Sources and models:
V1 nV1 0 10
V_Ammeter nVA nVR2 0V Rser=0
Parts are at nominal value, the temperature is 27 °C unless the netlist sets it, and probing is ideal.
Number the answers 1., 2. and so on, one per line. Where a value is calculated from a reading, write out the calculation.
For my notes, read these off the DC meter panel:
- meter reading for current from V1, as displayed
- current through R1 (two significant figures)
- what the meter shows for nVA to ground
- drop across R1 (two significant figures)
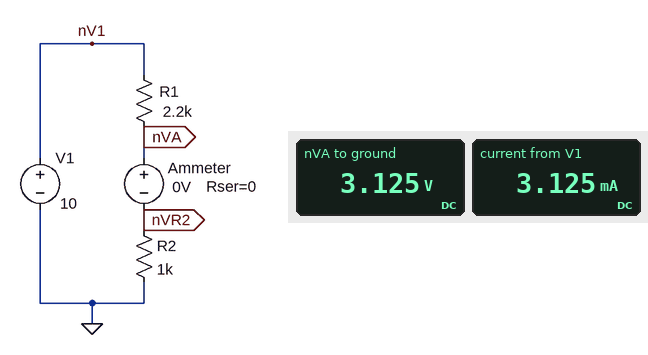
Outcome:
1. 3.125 mA
2. (10 V - 3.125 V) / 2.2 kΩ = 3.1 mA
3. 3.125 V
4. 10 V - 3.125 V = 6.9 V
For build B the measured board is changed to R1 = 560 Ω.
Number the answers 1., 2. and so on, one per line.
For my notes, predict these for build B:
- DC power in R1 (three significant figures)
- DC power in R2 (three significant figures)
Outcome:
1. 23.0 mW
2. 41.1 mW
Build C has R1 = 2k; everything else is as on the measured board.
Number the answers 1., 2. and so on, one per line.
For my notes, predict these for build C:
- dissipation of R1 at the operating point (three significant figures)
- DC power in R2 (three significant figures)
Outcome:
1. 22.2 mW
2. 11.1 mW
